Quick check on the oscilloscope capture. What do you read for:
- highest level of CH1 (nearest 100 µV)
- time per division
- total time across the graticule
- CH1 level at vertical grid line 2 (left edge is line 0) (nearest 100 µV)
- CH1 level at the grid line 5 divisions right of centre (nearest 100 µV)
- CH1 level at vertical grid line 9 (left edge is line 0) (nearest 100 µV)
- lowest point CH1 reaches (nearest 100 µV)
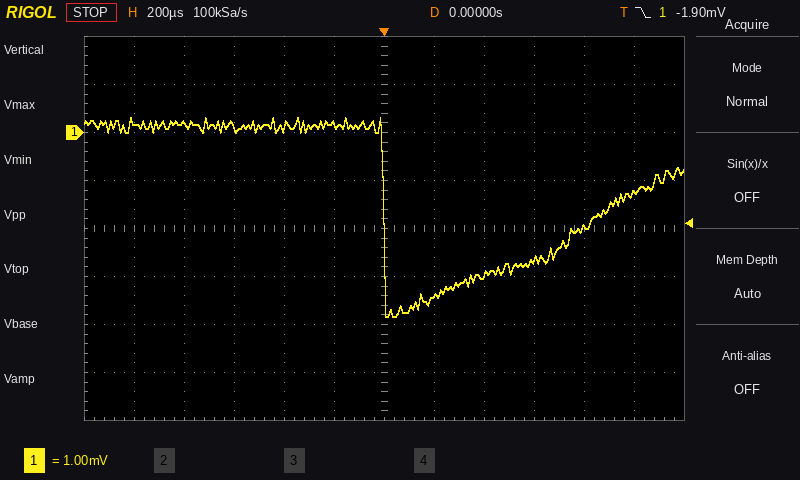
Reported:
300 µV
200 µs
2.4 ms
200 µV
-1.3 mV
-2.6 mV
-3.8 mV
